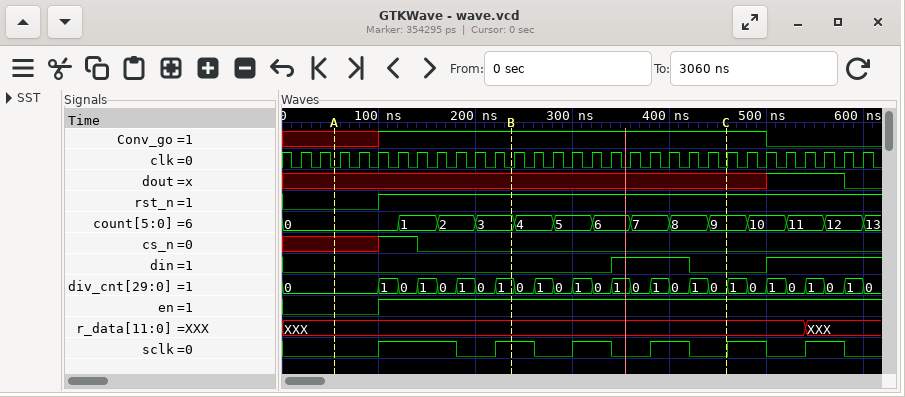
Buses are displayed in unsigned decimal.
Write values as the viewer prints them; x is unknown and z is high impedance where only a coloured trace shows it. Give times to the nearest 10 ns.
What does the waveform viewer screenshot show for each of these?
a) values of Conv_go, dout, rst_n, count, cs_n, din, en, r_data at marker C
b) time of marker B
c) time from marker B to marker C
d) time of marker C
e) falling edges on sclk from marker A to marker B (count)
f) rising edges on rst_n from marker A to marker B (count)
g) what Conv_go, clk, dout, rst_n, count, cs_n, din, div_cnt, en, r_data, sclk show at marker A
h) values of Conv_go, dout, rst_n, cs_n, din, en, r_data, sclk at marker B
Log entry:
Conv_go=1, dout=x, rst_n=1, count=9, cs_n=0, din=0, en=1, r_data=XXX
240 ns
220 ns
460 ns
1
1
Conv_go=x, clk=0, dout=x, rst_n=0, count=0, cs_n=x, din=0, div_cnt=0, en=0, r_data=XXX, sclk=0
Conv_go=1, dout=x, rst_n=1, cs_n=0, din=0, en=1, r_data=XXX, sclk=1
